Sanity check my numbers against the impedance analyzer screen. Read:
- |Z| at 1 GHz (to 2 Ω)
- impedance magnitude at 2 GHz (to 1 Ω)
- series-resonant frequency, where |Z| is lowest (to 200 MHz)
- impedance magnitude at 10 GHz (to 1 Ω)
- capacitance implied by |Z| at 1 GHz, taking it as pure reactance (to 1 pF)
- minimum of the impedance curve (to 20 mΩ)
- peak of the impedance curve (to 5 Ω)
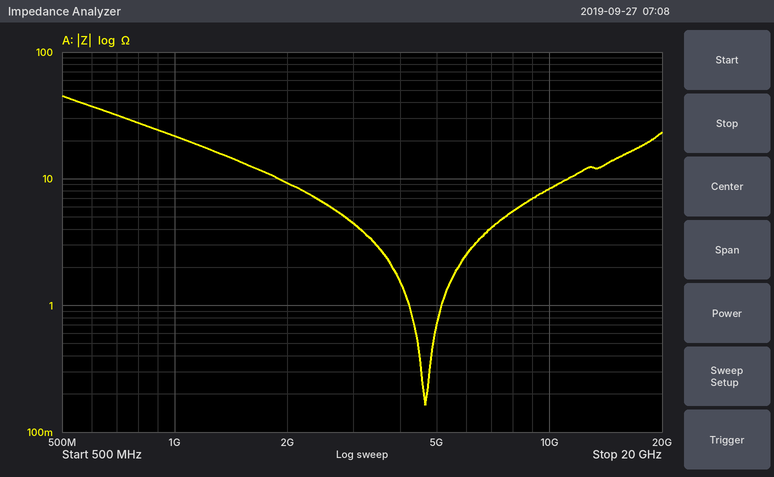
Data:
22 Ω
9 Ω
4.6 GHz
8 Ω
7 pF
160 mΩ
45 Ω
